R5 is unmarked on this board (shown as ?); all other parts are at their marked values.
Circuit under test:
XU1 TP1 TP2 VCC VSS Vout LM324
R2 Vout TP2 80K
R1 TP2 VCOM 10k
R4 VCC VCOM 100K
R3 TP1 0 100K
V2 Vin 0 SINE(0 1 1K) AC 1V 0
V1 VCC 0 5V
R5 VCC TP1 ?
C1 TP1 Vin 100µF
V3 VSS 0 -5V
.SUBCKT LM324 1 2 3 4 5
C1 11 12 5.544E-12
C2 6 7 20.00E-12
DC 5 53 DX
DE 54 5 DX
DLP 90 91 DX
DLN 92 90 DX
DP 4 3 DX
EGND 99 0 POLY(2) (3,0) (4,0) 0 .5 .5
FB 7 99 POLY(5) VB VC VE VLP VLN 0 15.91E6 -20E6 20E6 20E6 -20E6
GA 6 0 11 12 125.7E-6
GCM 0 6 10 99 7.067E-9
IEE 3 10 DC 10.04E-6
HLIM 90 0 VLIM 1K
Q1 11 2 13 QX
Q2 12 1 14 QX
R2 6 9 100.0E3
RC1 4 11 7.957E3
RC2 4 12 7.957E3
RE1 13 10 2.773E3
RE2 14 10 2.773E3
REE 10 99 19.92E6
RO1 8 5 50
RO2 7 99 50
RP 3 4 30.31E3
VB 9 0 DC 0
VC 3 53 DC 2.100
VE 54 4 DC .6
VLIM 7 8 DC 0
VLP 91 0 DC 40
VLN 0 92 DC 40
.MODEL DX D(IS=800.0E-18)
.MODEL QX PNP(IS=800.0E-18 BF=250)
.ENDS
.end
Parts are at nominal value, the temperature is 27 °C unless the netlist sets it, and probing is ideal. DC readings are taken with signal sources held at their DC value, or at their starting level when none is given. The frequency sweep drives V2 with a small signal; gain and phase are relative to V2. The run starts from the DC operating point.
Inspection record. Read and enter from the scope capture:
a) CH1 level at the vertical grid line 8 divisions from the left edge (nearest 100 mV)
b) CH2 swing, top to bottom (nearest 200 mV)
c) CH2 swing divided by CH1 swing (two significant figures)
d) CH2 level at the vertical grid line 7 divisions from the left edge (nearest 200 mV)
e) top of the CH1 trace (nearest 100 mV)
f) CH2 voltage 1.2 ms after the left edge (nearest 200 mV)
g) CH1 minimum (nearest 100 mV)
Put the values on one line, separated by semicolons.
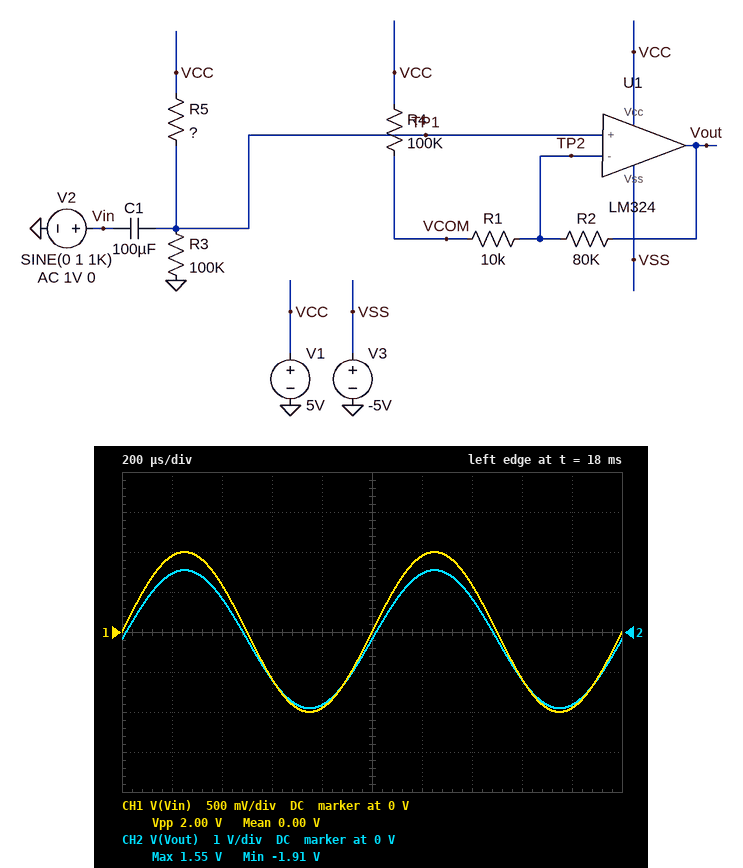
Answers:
-600 mV; 3.4 V; 1.7; 800 mV; 1.0 V; 1.4 V; -1.0 V
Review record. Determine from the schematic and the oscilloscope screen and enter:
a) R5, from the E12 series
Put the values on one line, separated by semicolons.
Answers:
150 kΩ
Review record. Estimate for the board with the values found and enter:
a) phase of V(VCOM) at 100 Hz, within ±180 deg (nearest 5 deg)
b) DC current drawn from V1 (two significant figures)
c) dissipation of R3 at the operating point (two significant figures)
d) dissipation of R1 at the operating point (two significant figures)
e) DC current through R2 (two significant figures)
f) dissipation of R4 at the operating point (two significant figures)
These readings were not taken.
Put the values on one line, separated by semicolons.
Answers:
0 deg; 390 µA; 40 µW; 7.4 µW; 27 µA; 74 µW
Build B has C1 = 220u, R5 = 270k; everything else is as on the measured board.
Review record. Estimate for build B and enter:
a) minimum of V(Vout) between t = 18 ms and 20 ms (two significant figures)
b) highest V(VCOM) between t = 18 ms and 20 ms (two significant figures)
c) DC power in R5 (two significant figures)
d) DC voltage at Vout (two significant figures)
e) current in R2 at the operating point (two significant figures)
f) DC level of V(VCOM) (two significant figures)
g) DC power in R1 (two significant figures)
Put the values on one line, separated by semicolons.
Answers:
-3.0 V; 2.6 V; 49 µW; -1.3 V; 33 µA; 1.7 V; 11 µW
